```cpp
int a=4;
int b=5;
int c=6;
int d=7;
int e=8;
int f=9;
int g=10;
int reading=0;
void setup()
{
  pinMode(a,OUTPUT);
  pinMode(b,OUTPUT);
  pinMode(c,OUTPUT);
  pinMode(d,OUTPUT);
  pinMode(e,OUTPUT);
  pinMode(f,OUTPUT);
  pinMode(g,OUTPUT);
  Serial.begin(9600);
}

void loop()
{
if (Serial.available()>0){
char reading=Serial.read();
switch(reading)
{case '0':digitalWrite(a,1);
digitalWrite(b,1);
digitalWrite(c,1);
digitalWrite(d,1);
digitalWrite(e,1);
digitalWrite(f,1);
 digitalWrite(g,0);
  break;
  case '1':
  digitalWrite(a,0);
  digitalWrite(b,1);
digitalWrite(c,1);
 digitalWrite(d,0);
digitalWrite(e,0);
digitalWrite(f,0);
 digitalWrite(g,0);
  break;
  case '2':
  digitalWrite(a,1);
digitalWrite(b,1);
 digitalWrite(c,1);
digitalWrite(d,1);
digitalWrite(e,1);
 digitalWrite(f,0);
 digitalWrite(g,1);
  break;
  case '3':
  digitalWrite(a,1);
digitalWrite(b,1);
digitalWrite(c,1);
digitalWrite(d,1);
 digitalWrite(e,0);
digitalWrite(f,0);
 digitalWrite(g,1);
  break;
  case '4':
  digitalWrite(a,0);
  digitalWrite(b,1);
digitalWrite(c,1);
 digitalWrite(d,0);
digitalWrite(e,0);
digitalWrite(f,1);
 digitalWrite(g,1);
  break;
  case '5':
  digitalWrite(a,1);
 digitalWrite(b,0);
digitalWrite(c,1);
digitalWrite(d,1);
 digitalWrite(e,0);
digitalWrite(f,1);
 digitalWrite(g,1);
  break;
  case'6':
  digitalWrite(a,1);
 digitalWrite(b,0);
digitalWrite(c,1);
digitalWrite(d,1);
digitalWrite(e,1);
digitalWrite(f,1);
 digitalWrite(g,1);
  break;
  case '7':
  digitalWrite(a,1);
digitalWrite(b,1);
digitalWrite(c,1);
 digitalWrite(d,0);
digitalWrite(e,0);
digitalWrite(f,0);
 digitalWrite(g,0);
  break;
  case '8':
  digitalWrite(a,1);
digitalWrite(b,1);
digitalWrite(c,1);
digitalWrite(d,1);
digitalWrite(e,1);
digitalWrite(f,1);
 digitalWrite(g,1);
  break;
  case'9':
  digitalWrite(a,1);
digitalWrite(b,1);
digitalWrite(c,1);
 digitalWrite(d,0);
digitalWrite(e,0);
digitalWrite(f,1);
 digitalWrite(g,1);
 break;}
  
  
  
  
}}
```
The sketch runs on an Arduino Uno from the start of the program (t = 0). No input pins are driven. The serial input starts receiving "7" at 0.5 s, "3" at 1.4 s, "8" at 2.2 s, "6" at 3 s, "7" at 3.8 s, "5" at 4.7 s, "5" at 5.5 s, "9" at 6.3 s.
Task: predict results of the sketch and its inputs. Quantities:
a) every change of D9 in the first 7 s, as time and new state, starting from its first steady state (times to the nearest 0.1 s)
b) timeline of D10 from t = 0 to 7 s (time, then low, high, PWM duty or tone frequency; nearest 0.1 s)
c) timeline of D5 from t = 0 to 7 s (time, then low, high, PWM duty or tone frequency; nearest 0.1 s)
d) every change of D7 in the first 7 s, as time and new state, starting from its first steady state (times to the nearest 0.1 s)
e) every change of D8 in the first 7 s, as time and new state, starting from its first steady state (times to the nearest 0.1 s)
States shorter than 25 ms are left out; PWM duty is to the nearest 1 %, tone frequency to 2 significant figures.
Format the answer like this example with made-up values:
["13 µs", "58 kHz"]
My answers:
["0 s low; 2.2 s high; 3.8 s low; 4.7 s high", "0 s low; 1.4 s high; 3.8 s low; 4.7 s high", "0 s low; 0.5 s high; 3 s low; 3.8 s high; 4.7 s low; 6.3 s high", "0 s low; 1.4 s high; 3.8 s low; 4.7 s high; 6.3 s low", "0 s low; 2.2 s high; 3.8 s low"]
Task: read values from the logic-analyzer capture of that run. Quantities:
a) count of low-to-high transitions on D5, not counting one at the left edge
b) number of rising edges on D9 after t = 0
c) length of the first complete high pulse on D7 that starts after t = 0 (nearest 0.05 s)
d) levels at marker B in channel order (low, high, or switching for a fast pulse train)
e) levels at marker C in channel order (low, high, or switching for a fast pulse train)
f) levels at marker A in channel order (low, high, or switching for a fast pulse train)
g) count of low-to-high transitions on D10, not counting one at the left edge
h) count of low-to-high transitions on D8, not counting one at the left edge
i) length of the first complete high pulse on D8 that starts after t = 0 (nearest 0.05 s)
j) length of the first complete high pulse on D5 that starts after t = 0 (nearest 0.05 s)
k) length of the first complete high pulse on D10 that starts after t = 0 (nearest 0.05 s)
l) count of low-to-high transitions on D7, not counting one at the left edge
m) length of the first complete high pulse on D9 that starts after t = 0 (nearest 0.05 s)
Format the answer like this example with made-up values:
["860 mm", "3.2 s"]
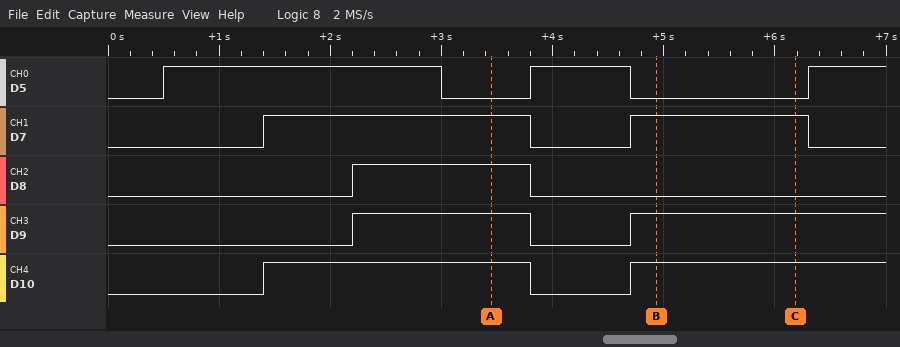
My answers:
["3", "2", "2.40 s", "D5 low, D7 high, D8 low, D9 high, D10 high", "D5 low, D7 high, D8 low, D9 high, D10 high", "D5 low, D7 high, D8 high, D9 high, D10 high", "2", "1", "1.60 s", "2.50 s", "2.40 s", "2", "1.60 s"]
